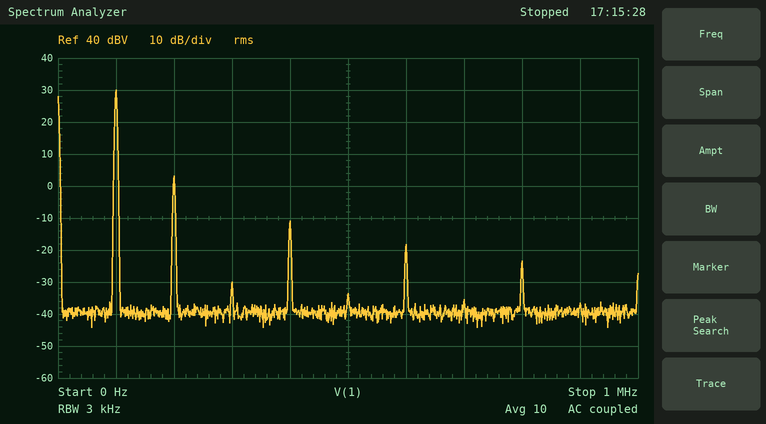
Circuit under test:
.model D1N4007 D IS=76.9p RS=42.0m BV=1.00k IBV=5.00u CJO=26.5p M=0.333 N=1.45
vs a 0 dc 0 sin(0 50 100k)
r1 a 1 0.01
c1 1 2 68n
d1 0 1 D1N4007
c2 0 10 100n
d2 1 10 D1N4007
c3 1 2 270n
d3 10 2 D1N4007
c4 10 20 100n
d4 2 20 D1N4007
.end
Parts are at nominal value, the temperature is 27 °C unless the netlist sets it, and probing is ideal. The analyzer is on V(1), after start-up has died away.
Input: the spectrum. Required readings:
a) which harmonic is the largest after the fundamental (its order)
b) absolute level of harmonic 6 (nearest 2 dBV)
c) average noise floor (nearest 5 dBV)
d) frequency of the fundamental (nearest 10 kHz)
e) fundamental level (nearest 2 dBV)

2
-18 dBV
-40 dBV
100 kHz
30 dBV
